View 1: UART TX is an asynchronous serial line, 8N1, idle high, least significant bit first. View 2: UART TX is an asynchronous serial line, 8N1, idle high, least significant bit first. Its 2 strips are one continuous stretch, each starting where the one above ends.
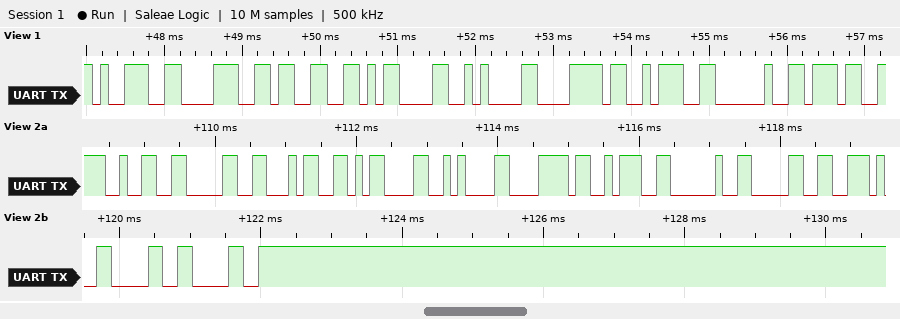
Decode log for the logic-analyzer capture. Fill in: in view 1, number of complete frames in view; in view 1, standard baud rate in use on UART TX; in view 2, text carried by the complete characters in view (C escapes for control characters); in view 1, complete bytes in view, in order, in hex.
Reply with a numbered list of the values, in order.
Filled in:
1. 9
2. 9600 baud
3. "204\r\nx: 0.00"
4. 39 38 33 0D 0A 78 3A 20 37
